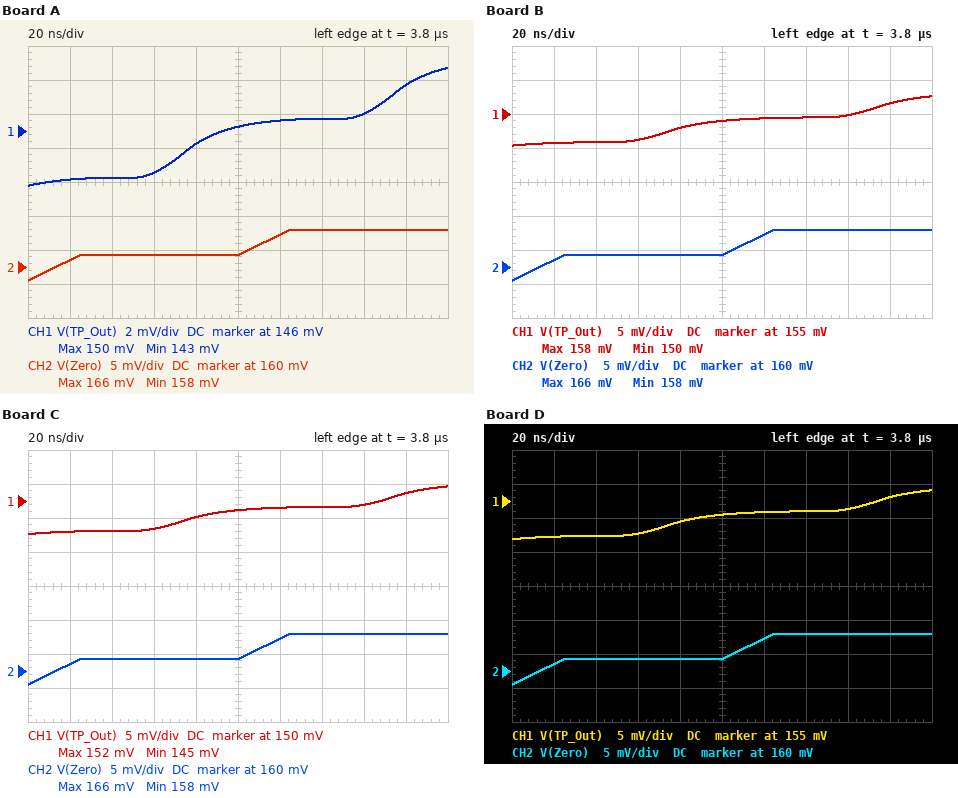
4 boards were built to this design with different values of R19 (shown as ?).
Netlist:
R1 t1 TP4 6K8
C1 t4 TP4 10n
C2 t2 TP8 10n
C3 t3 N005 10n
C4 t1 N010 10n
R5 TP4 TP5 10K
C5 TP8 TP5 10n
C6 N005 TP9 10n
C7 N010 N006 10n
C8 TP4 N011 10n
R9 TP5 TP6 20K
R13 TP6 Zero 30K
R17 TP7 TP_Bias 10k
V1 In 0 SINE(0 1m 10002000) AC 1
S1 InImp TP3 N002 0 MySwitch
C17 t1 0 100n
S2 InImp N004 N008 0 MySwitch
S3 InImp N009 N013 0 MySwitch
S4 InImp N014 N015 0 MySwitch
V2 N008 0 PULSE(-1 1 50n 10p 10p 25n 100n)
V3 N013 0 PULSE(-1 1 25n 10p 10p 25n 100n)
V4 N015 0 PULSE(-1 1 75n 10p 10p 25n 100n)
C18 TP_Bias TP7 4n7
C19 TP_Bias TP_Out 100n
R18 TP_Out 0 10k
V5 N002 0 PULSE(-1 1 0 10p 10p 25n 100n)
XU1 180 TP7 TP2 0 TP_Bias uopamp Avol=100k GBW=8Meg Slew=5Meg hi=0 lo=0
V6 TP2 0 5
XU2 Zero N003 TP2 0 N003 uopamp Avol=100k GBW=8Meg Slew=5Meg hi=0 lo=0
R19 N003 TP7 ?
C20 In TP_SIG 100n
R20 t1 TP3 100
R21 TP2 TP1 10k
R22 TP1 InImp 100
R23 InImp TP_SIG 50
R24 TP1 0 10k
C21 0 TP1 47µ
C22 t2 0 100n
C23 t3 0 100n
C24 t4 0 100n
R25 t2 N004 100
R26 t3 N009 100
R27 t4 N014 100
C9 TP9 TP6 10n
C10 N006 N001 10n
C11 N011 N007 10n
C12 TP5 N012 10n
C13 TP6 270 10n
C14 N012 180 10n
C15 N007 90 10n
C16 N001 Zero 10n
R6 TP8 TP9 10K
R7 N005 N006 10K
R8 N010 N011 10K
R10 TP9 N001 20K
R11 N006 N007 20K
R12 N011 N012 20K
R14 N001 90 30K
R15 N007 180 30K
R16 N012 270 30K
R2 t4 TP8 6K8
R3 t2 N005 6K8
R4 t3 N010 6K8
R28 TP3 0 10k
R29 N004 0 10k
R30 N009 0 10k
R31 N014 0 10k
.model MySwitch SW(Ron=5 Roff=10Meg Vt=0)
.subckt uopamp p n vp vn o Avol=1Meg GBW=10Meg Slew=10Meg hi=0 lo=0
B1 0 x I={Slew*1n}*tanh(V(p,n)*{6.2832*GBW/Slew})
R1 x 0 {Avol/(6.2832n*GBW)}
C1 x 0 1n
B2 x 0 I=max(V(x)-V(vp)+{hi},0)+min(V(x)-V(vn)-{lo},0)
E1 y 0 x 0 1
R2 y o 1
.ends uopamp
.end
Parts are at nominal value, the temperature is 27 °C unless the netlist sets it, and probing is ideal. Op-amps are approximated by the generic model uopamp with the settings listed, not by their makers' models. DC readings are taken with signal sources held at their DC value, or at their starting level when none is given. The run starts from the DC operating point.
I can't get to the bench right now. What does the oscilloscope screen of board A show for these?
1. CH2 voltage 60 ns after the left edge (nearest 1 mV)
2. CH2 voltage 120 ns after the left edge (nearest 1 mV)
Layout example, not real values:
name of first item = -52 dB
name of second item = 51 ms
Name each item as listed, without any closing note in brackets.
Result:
CH2 voltage 60 ns after the left edge = 162 mV
CH2 voltage 120 ns after the left edge = 165 mV
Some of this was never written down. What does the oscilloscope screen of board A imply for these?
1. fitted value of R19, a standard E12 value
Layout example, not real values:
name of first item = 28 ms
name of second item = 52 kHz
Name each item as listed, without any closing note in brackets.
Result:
fitted value of R19, a standard E12 value = 120 Ω
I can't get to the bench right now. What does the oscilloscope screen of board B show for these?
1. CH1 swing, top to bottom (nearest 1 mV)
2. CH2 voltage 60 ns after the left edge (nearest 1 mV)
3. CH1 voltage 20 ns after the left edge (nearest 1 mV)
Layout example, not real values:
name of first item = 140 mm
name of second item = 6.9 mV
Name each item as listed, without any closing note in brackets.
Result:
CH1 swing, top to bottom = 7 mV
CH2 voltage 60 ns after the left edge = 162 mV
CH1 voltage 20 ns after the left edge = 151 mV
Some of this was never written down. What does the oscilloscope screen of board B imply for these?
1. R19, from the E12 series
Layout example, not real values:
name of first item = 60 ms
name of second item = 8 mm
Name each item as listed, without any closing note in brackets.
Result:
R19, from the E12 series = 330 Ω
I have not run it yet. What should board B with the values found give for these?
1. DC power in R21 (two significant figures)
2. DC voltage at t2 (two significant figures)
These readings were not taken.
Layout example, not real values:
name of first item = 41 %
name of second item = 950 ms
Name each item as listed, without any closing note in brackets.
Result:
DC power in R21 = 630 µW
DC voltage at t2 = 2.5 mV
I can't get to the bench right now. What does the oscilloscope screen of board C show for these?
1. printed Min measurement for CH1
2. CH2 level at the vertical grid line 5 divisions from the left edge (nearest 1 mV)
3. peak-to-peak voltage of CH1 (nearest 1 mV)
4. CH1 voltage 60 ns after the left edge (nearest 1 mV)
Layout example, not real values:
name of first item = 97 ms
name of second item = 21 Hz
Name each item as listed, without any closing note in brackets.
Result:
printed Min measurement for CH1 = 145 mV
CH2 level at the vertical grid line 5 divisions from the left edge = 162 mV
peak-to-peak voltage of CH1 = 7 mV
CH1 voltage 60 ns after the left edge = 146 mV
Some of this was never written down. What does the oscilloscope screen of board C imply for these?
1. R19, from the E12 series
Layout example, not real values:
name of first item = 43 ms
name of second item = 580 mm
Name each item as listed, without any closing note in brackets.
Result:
R19, from the E12 series = 150 Ω
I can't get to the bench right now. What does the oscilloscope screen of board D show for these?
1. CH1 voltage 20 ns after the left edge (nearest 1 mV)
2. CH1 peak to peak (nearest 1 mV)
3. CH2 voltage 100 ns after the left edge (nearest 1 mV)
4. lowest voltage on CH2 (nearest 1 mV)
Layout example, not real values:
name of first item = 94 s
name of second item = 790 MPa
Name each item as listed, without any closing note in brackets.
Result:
CH1 voltage 20 ns after the left edge = 150 mV
CH1 peak to peak = 7 mV
CH2 voltage 100 ns after the left edge = 162 mV
lowest voltage on CH2 = 158 mV
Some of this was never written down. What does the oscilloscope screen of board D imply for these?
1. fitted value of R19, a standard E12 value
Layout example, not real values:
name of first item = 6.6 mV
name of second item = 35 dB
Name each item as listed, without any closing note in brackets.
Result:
fitted value of R19, a standard E12 value = 270 Ω
